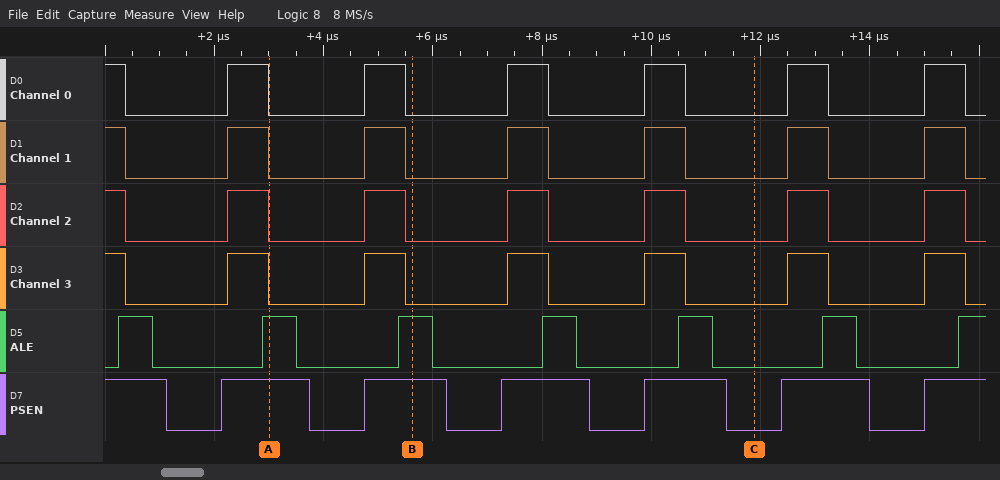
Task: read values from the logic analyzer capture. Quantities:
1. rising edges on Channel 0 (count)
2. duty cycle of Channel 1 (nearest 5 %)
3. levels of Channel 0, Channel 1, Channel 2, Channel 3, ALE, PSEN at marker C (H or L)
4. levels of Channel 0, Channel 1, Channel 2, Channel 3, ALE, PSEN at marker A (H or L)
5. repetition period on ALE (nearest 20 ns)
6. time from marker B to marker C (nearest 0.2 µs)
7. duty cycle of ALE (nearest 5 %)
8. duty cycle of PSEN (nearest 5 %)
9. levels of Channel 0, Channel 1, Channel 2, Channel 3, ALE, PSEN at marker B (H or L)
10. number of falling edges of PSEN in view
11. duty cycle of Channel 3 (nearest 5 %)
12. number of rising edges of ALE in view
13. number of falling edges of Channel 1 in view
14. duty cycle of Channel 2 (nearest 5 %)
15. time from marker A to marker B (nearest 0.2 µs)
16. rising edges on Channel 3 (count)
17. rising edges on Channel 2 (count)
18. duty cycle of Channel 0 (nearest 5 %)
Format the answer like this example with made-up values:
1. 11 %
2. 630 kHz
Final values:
1. 6
2. 30 %
3. Channel 0=L, Channel 1=L, Channel 2=L, Channel 3=L, ALE=L, PSEN=L
4. Channel 0=L, Channel 1=L, Channel 2=L, Channel 3=L, ALE=H, PSEN=H
5. 2560 ns
6. 6.2 µs
7. 25 %
8. 60 %
9. Channel 0=L, Channel 1=L, Channel 2=L, Channel 3=L, ALE=H, PSEN=H
10. 6
11. 30 %
12. 7
13. 7
14. 30 %
15. 2.6 µs
16. 6
17. 6
18. 30 %
